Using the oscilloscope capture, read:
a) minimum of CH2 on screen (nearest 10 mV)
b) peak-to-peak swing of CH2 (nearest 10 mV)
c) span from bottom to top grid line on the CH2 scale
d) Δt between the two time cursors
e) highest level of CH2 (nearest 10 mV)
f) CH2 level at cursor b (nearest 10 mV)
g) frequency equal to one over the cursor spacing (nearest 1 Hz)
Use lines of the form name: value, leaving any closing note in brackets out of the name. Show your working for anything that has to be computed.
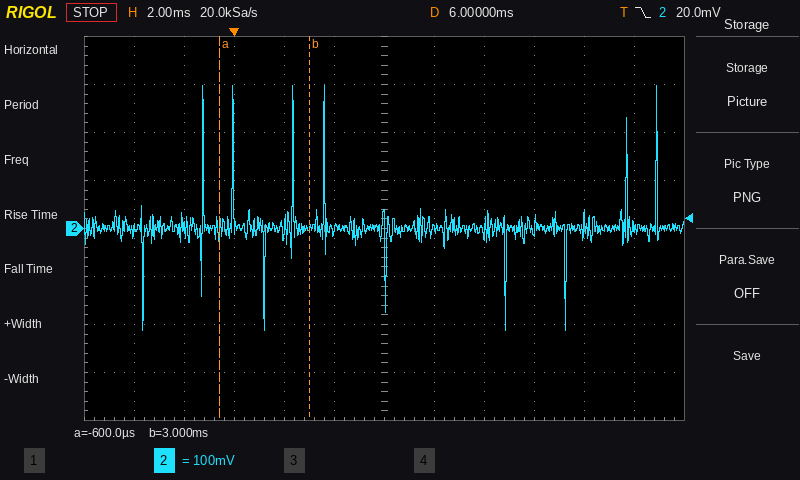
minimum of CH2 on screen: -210 mV
peak-to-peak swing of CH2: 300 mV − (-210 mV) = 510 mV
span from bottom to top grid line on the CH2 scale: 800 mV
Δt between the two time cursors: 3 ms − (-600 µs) = 3.6 ms
highest level of CH2: 300 mV
CH2 level at cursor b: 0 mV
frequency equal to one over the cursor spacing: 1 / 3.6 ms ≈ 278 Hz
